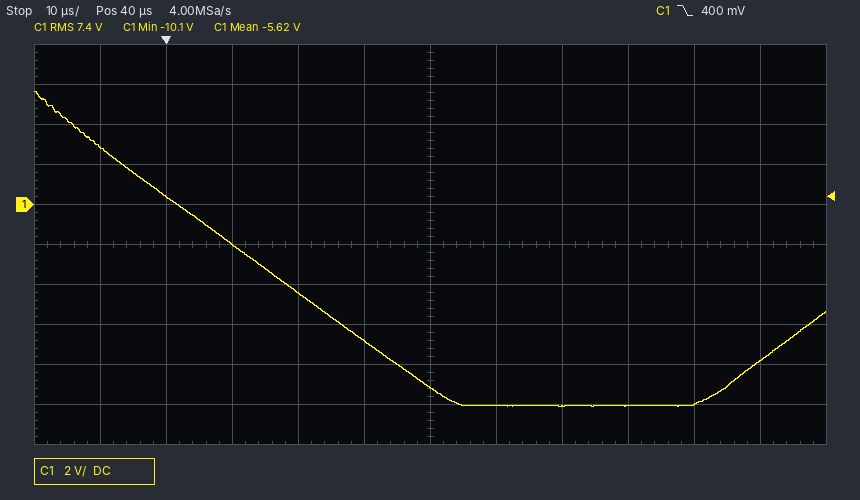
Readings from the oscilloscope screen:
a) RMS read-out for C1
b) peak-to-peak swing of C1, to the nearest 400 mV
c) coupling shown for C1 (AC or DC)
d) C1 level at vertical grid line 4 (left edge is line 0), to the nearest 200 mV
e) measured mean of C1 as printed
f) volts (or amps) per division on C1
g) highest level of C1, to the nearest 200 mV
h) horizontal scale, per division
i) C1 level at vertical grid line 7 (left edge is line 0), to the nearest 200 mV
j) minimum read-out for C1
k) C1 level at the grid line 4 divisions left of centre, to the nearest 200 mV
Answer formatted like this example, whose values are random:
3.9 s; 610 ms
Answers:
7.4 V; 15.6 V; DC; -4.4 V; -5.62 V; 2 V; 5.6 V; 10 µs; -10.0 V; -10.1 V; 400 mV
